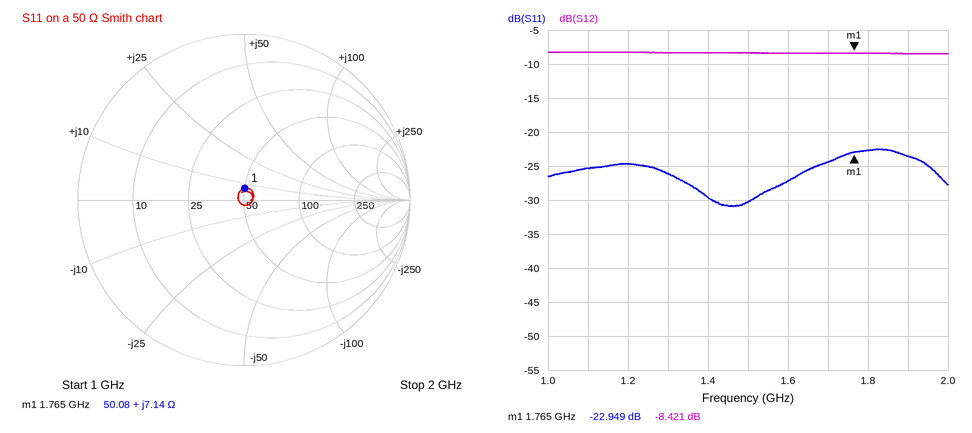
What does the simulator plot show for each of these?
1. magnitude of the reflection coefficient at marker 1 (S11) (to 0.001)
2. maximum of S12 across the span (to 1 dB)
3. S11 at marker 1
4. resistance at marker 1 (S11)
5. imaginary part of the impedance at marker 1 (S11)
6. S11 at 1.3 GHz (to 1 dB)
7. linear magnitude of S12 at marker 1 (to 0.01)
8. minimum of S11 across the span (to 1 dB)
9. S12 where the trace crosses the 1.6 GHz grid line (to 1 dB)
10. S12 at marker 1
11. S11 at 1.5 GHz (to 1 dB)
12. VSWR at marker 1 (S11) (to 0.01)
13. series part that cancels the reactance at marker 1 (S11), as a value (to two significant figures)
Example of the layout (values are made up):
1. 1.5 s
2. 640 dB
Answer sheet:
1. 0.071
2. -8 dB
3. -22.949 dB
4. 50.08 Ω
5. +7.14 Ω
6. -26 dB
7. 0.38
8. -31 dB
9. -8 dB
10. -8.421 dB
11. -30 dB
12. 1.15
13. 13 pF
